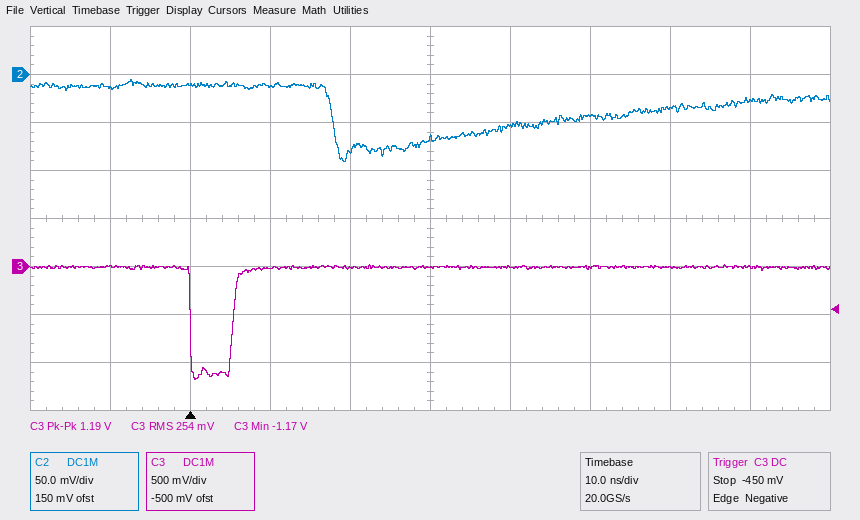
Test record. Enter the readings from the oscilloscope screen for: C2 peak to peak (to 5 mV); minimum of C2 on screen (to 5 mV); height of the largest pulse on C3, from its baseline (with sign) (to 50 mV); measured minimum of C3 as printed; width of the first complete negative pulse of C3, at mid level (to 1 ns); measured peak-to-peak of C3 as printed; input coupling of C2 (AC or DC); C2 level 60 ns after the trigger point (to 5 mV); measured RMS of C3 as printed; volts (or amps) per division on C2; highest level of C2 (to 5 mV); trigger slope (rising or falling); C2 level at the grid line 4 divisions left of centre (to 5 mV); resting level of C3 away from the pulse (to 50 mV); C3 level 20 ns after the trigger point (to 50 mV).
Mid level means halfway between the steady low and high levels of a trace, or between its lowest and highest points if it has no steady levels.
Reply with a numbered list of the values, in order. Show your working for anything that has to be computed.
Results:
1. -5 mV − (-90 mV) = 85 mV
2. -90 mV
3. -1.15 V
4. -1.17 V
5. 5 ns
6. 1.19 V
7. DC
8. -35 mV
9. 254 mV
10. 50 mV
11. -5 mV
12. falling
13. -15 mV
14. 0 mV
15. 0 mV
